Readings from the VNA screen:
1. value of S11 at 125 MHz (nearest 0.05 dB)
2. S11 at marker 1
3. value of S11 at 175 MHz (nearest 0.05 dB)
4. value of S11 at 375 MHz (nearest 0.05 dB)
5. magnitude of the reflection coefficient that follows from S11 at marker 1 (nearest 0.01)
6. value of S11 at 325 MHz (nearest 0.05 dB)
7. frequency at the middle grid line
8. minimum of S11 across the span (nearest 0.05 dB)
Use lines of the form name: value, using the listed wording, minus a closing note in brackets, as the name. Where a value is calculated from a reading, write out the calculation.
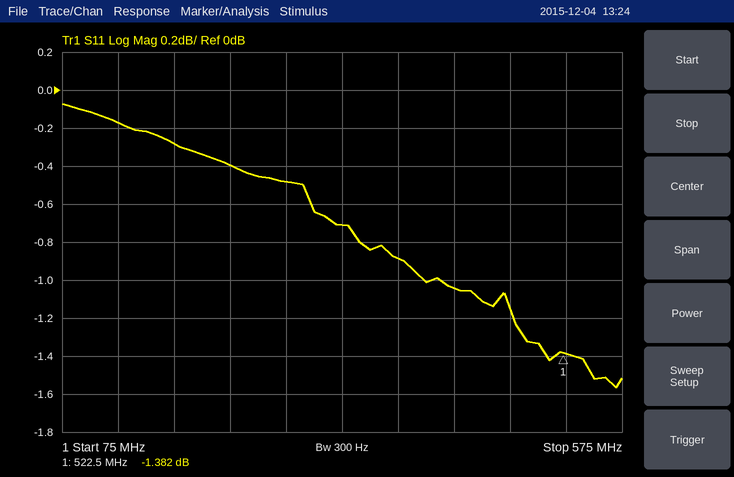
value of S11 at 125 MHz: -0.15 dB
S11 at marker 1: -1.382 dB
value of S11 at 175 MHz: -0.30 dB
value of S11 at 375 MHz: -0.90 dB
magnitude of the reflection coefficient that follows from S11 at marker 1: 10^(-1.382/20) ≈ 0.85
value of S11 at 325 MHz: -0.70 dB
frequency at the middle grid line: 325 MHz
minimum of S11 across the span: -1.55 dB
